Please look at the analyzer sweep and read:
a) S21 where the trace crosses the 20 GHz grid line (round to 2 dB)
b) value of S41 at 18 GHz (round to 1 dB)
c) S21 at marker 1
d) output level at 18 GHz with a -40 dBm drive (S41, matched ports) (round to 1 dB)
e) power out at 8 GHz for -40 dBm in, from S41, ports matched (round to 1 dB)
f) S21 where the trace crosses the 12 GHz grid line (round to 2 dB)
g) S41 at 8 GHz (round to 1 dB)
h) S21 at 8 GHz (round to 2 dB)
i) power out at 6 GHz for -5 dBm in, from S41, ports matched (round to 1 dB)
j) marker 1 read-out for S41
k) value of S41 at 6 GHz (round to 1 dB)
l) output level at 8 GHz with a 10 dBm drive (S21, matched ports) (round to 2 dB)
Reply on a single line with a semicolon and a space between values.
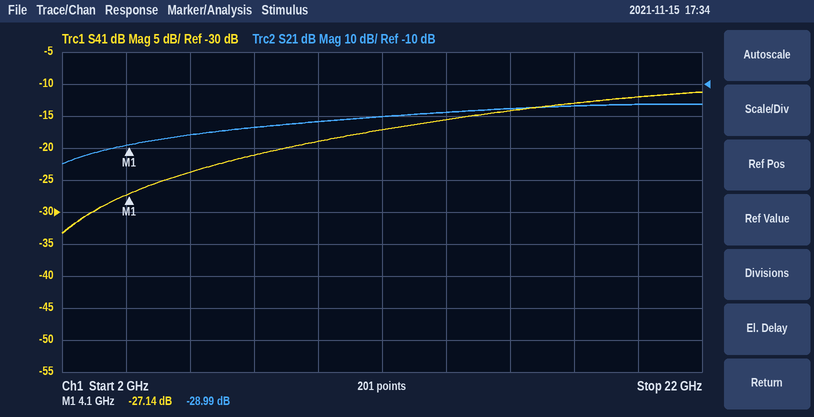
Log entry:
-16 dB; -13 dB; -28.99 dB; -53 dBm; -61 dBm; -20 dB; -21 dB; -24 dB; -29 dBm; -27.14 dB; -24 dB; -14 dBm
